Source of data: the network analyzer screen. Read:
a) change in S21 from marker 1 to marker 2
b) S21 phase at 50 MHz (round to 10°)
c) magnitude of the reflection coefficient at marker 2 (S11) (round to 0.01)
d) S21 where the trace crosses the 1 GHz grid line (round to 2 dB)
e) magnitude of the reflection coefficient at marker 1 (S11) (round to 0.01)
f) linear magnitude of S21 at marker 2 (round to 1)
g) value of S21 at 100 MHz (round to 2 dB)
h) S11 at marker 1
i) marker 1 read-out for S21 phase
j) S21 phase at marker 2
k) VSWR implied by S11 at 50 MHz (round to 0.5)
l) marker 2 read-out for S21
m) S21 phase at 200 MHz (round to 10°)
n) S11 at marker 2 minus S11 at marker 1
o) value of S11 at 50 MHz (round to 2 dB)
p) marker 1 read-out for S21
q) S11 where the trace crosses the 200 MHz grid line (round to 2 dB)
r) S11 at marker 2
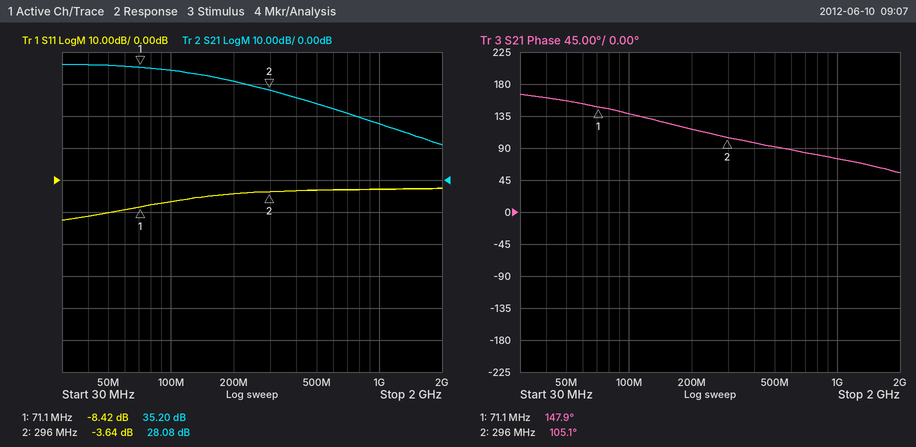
-7.12 dB
160°
0.66
18 dB
0.38
25
34 dB
-8.42 dB
147.9°
105.1°
2.0
28.08 dB
120°
4.78 dB
-10 dB
35.20 dB
-4 dB
-3.64 dB
